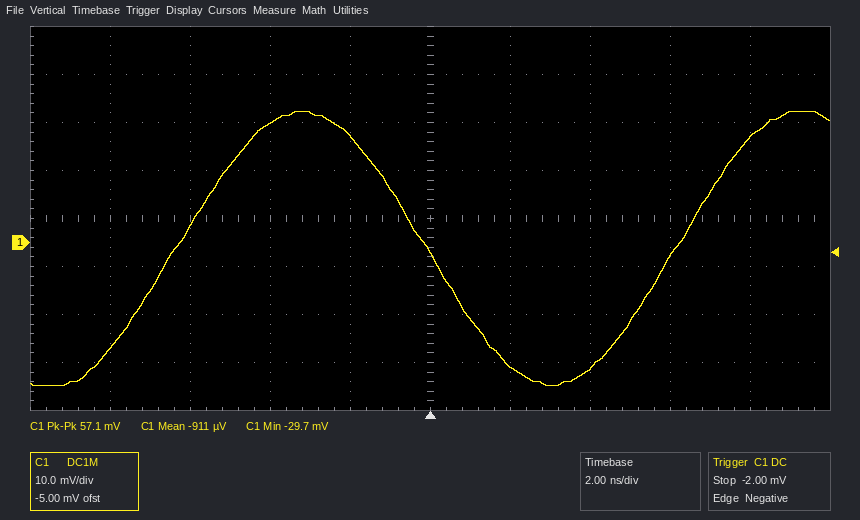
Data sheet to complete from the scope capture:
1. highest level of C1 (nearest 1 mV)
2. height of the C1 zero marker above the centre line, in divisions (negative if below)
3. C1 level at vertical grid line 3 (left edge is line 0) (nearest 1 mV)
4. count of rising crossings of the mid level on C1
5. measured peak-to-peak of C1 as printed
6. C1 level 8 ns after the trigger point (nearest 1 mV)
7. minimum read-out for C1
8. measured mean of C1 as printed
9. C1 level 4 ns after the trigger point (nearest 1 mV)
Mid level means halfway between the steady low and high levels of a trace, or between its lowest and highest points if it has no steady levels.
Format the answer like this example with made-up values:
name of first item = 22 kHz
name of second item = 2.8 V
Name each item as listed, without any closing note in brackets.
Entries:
highest level of C1 = 27 mV
height of the C1 zero marker above the centre line, in divisions = -0.5 div
C1 level at vertical grid line 3 (left edge is line 0) = 25 mV
count of rising crossings of the mid level on C1 = 2
measured peak-to-peak of C1 as printed = 57.1 mV
C1 level 8 ns after the trigger point = 22 mV
minimum read-out for C1 = -29.7 mV
measured mean of C1 as printed = -911 µV
C1 level 4 ns after the trigger point = -26 mV
